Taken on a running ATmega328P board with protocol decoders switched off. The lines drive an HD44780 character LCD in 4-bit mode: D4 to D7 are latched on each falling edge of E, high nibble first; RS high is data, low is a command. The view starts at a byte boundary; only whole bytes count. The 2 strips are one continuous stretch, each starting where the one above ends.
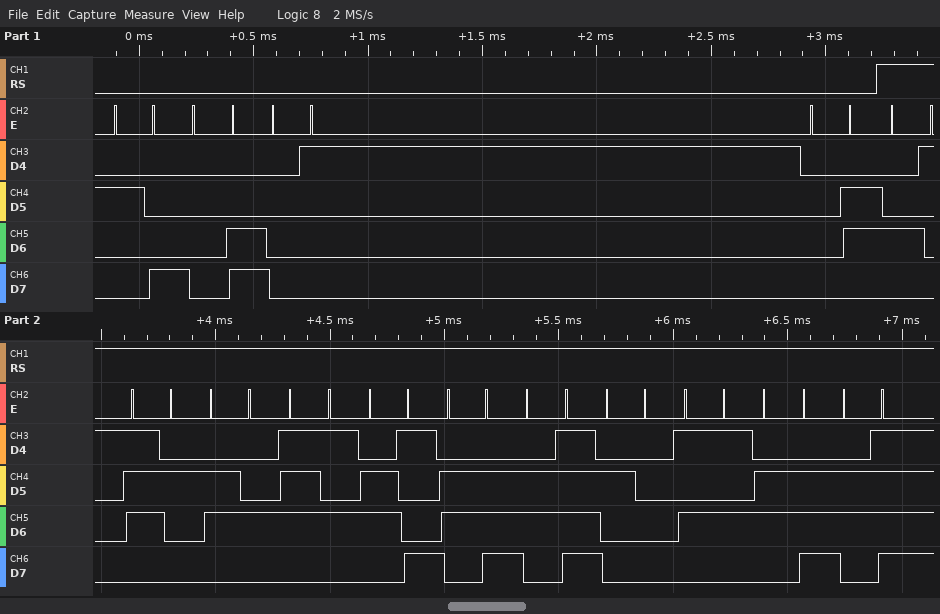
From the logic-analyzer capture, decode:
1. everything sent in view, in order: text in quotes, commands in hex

0x28 0x0C 0x01 0x06 "Arduino Uno"
